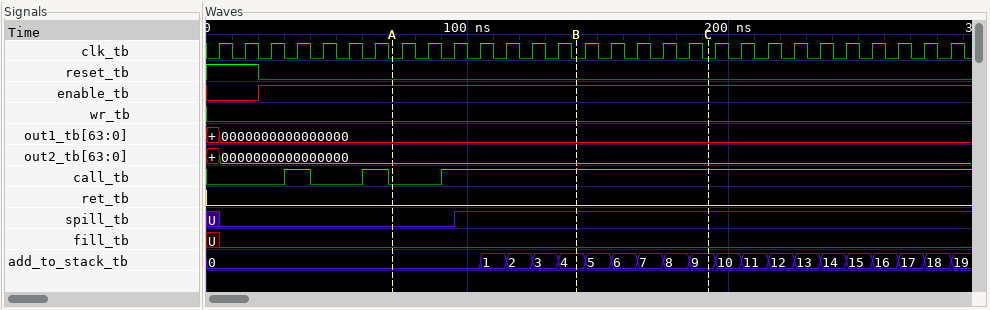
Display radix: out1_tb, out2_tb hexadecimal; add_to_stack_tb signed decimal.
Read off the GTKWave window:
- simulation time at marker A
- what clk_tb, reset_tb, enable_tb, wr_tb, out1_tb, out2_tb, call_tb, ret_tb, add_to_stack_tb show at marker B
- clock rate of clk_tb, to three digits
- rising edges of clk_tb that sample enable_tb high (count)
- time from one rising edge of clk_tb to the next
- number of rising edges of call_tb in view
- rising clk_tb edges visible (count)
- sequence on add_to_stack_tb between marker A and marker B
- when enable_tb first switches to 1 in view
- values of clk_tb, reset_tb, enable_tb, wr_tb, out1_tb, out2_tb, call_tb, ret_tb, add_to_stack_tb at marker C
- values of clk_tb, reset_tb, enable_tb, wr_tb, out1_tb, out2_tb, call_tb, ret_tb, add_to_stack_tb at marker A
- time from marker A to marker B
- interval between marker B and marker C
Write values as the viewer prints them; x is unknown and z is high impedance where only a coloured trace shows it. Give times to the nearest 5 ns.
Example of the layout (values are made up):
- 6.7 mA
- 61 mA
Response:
- 70 ns
- clk_tb=0, reset_tb=0, enable_tb=1, wr_tb=0, out1_tb=0000000000000000, out2_tb=0000000000000000, call_tb=1, ret_tb=0, add_to_stack_tb=4
- 100 MHz
- 27
- 10 ns
- 3
- 29
- 0, 1, 2, 3, 4
- 20 ns
- clk_tb=0, reset_tb=0, enable_tb=1, wr_tb=0, out1_tb=0000000000000000, out2_tb=0000000000000000, call_tb=1, ret_tb=0, add_to_stack_tb=9
- clk_tb=0, reset_tb=0, enable_tb=1, wr_tb=0, out1_tb=0000000000000000, out2_tb=0000000000000000, call_tb=0, ret_tb=0, add_to_stack_tb=0
- 70 ns
- 50 ns
